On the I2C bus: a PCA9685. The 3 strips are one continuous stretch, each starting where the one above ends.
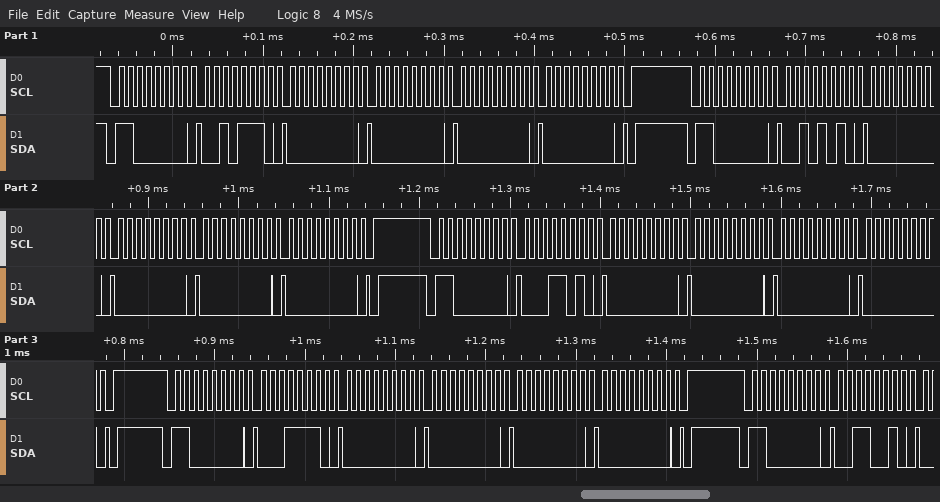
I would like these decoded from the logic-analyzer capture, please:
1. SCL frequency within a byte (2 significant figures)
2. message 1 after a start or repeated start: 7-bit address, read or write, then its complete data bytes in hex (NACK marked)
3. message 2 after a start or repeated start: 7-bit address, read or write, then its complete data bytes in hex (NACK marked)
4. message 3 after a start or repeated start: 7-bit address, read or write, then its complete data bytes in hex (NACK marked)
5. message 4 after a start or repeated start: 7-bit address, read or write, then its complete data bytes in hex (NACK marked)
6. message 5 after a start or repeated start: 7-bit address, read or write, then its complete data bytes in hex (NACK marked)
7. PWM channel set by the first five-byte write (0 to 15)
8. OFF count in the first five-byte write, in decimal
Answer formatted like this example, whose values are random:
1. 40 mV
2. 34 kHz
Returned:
1. 100 kHz
2. 0x60 write: 2E 00 00 00 00
3. 0x60 write: 2A 00 00 00 00
4. 0x60 write: 1A 00 00 00 00
5. 0x60 write: 1E 00 00 00 00
6. 0x60 write: 32
7. 10
8. 0
